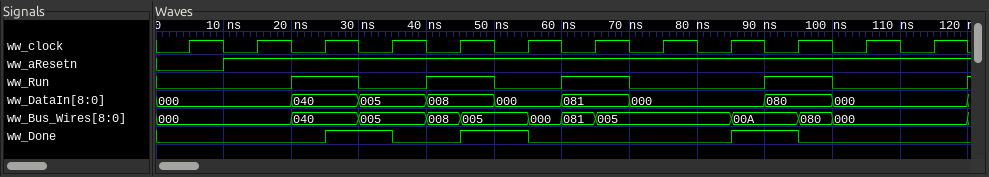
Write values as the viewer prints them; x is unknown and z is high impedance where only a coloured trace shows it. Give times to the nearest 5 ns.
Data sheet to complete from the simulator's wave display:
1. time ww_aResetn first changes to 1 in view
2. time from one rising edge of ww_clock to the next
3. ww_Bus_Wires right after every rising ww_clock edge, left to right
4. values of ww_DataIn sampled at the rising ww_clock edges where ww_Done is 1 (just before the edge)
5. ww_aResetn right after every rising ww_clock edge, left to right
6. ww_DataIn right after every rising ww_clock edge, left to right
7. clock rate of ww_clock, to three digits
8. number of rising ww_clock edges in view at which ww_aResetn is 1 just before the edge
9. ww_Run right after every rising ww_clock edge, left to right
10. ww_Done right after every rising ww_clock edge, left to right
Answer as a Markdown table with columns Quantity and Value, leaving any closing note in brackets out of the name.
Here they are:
| Quantity | Value |
|---|---|
| time ww_aResetn first changes to 1 in view | 10 ns |
| time from one rising edge of ww_clock to the next | 10 ns |
| ww_Bus_Wires right after every rising ww_clock edge, left to right | 000, 000, 040, 005, 005, 000, 005, 005, 00A, 080, 000, 000 |
| values of ww_DataIn sampled at the rising ww_clock edges where ww_Done is 1 | 005, 000, 080 |
| ww_aResetn right after every rising ww_clock edge, left to right | 0 1 1 1 1 1 1 1 1 1 1 1 |
| ww_DataIn right after every rising ww_clock edge, left to right | 000, 000, 040, 005, 008, 000, 081, 000, 000, 080, 000, 000 |
| clock rate of ww_clock, to three digits | 100 MHz |
| number of rising ww_clock edges in view at which ww_aResetn is 1 just before the edge | 11 |
| ww_Run right after every rising ww_clock edge, left to right | 0 0 1 0 1 0 1 0 0 1 0 0 |
| ww_Done right after every rising ww_clock edge, left to right | 0 0 1 0 1 0 0 0 1 0 0 0 |
